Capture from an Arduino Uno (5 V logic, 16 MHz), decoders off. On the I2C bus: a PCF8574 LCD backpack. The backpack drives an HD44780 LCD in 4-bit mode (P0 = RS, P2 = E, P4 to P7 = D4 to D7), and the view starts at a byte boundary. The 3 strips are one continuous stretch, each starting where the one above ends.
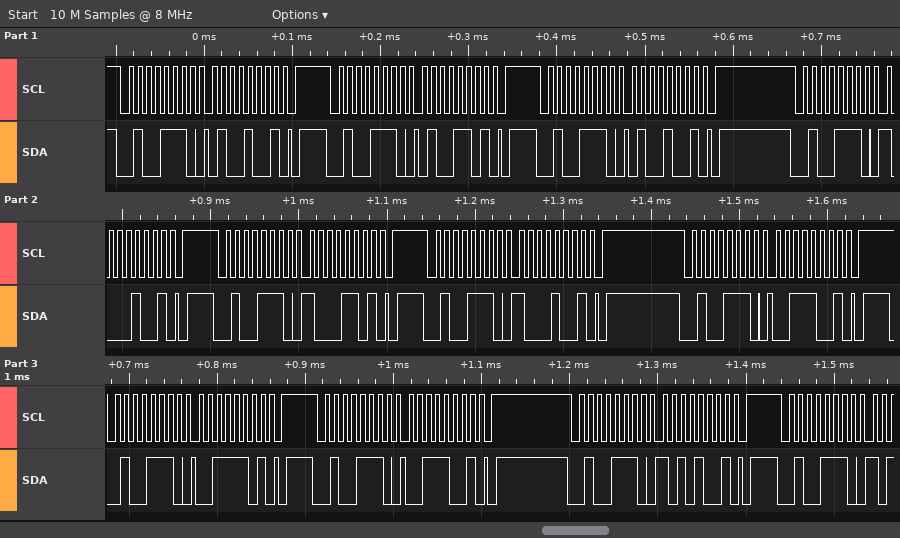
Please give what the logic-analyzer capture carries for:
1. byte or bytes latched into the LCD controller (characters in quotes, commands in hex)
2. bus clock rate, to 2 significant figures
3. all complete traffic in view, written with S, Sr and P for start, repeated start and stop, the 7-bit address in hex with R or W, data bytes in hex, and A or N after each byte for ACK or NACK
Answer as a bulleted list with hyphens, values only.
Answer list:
- 'H'
- 100 kHz
- S 27W A 49 A P S 27W A 4D A P S 27W A 49 A P S 27W A 89 A P S 27W A 8D A P S 27W A 89 A P S 27W A 39 A P S 27W A 3D A P S 27W A 39 A P S 27W A A9 A P S 27W A
